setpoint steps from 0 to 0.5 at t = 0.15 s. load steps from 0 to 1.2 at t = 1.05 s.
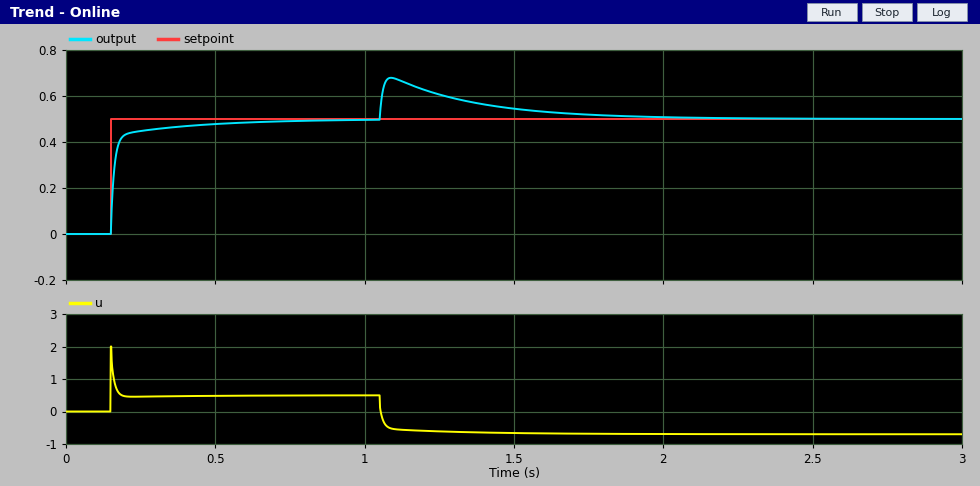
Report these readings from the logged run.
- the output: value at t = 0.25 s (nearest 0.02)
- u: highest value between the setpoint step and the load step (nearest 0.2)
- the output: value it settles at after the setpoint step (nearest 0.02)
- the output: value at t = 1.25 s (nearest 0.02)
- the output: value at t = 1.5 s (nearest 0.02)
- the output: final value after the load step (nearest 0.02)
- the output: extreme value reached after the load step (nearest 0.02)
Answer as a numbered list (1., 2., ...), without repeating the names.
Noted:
1. 0.44
2. 2.0
3. 0.50
4. 0.60
5. 0.54
6. 0.50
7. 0.68
